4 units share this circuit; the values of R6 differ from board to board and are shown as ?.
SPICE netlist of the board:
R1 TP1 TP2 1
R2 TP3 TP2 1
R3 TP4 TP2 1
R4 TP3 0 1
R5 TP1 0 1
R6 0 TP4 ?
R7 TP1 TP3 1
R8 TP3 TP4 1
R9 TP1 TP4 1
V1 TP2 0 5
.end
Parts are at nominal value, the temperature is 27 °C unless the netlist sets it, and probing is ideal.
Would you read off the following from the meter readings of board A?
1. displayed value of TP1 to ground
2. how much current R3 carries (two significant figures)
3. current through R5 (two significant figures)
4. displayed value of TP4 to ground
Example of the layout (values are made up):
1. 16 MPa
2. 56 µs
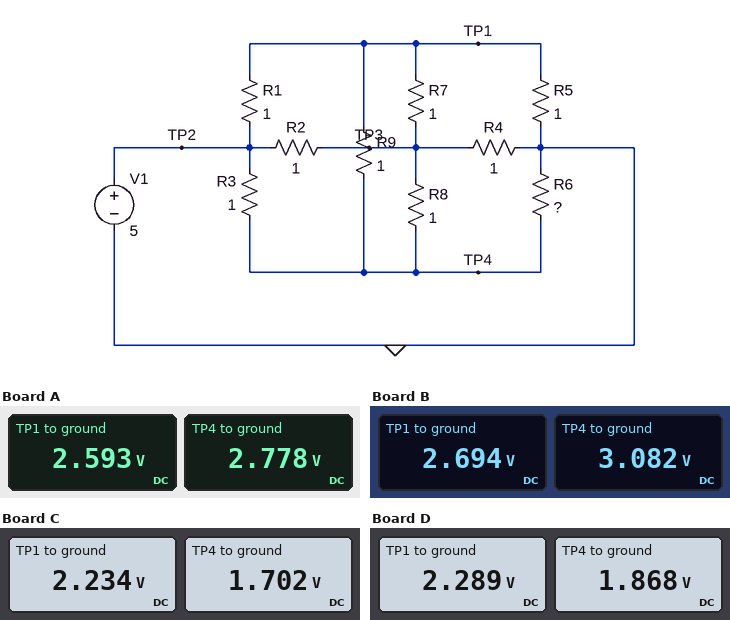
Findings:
1. 2.593 V
2. 2.2 A
3. 2.6 A
4. 2.778 V
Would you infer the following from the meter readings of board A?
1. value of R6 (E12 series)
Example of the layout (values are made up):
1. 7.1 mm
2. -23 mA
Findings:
1. 1.5 Ω
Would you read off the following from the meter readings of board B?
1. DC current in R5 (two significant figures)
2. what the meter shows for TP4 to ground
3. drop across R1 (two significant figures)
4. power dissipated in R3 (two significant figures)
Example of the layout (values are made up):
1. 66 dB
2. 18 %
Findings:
1. 2.7 A
2. 3.082 V
3. 2.3 V
4. 3.7 W
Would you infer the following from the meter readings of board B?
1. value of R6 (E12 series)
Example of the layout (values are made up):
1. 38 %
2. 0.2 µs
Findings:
1. 2.7 Ω
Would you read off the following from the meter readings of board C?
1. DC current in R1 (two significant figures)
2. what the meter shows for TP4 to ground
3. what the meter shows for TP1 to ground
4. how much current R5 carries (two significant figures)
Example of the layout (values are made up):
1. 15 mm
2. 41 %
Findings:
1. 2.8 A
2. 1.702 V
3. 2.234 V
4. 2.2 A
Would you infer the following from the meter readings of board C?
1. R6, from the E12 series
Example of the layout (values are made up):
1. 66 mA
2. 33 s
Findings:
1. 0.39 Ω
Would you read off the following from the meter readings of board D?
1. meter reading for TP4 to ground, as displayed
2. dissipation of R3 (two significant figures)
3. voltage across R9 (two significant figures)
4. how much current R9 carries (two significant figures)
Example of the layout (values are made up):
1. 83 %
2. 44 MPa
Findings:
1. 1.868 V
2. 9.8 W
3. 420 mV
4. 420 mA
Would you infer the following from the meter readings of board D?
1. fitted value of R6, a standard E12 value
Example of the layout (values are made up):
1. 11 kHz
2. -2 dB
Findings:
1. 0.47 Ω
